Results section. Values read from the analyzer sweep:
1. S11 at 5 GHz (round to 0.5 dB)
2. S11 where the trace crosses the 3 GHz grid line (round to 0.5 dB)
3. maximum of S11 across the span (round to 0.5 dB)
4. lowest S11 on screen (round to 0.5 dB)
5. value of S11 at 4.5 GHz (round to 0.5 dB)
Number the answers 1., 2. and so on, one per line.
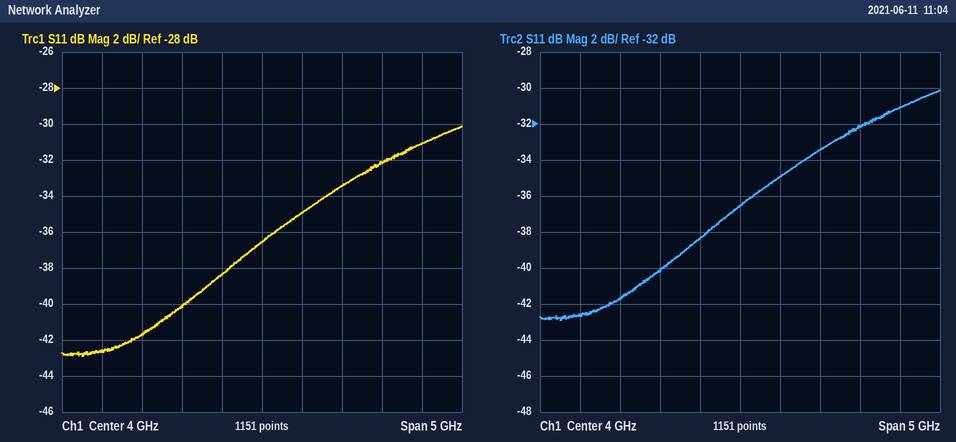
1. -33.5 dB
2. -40.0 dB
3. -30.0 dB
4. -43.0 dB
5. -35.0 dB
